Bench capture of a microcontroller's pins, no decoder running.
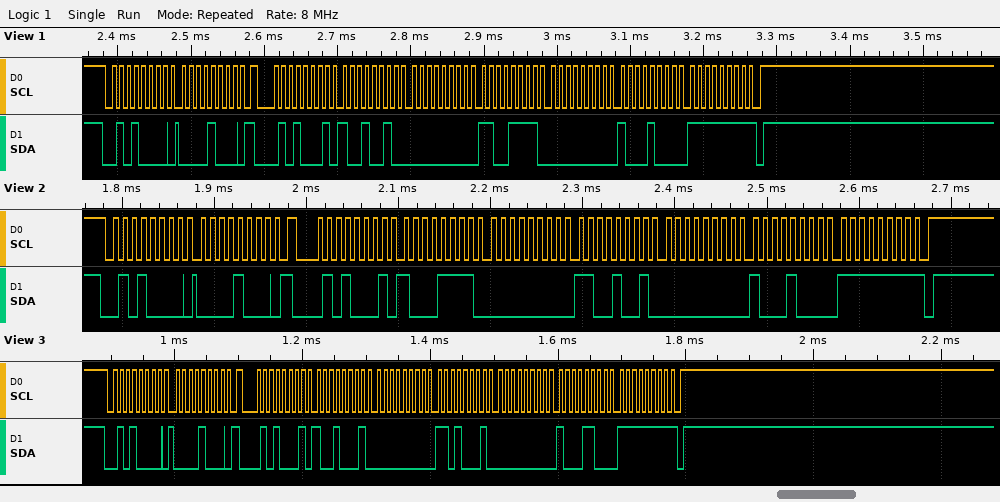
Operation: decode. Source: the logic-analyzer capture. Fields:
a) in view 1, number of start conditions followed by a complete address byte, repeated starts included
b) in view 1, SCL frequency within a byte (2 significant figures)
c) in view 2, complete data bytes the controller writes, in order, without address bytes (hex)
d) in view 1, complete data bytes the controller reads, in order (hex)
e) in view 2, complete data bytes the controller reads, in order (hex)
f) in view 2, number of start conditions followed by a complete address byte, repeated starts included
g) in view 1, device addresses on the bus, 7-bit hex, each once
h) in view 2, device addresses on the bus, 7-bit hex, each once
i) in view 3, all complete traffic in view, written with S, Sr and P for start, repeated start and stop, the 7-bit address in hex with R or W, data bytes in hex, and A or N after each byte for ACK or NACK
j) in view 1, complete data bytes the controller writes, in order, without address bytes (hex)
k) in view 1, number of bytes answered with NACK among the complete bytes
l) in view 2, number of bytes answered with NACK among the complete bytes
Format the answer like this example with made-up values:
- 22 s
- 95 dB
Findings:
- 2
- 100 kHz
- 08
- 92 00 CF 00 88 FF
- 8F 00 C9 00 88 FF
- 2
- 0x28
- 0x28
- S 28W A 08 A Sr 28R A 91 A 00 A D1 A 00 A 8C A FF N P
- 08
- 1
- 1
